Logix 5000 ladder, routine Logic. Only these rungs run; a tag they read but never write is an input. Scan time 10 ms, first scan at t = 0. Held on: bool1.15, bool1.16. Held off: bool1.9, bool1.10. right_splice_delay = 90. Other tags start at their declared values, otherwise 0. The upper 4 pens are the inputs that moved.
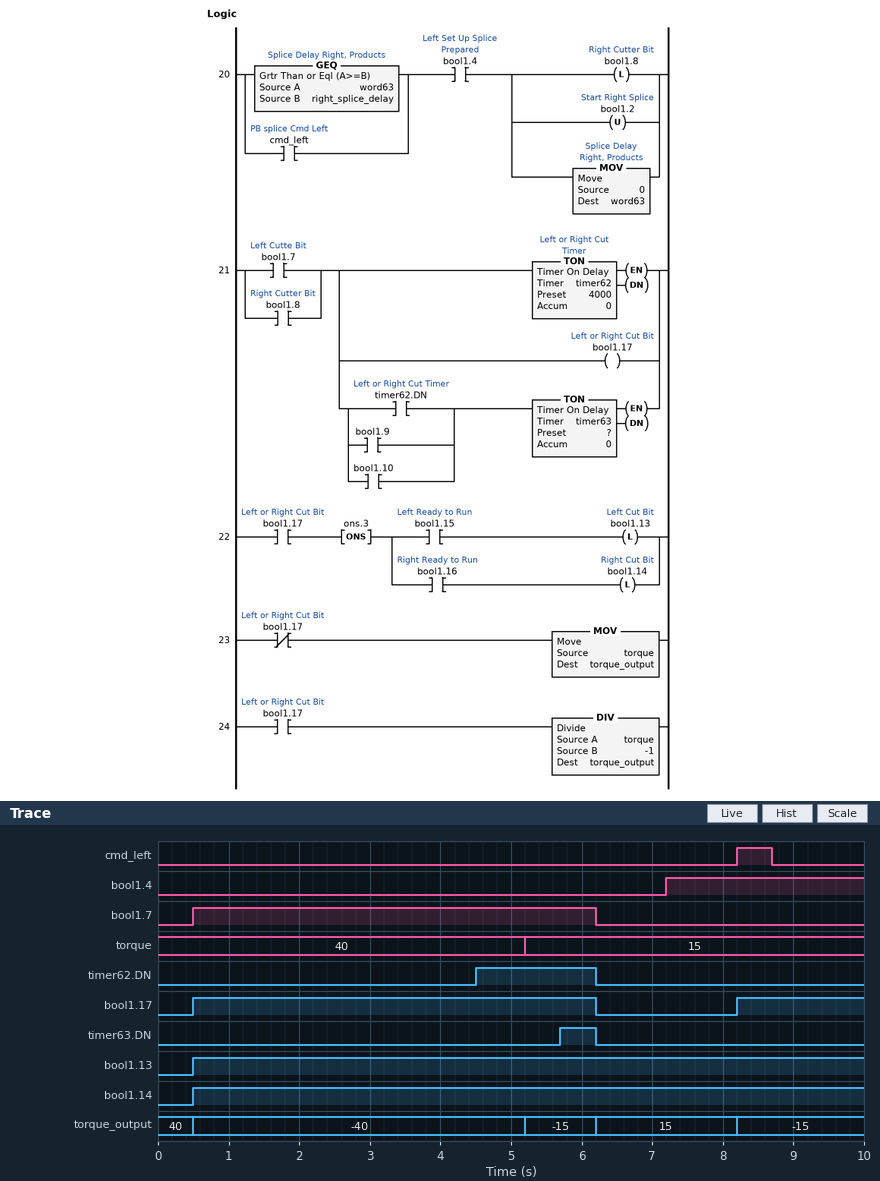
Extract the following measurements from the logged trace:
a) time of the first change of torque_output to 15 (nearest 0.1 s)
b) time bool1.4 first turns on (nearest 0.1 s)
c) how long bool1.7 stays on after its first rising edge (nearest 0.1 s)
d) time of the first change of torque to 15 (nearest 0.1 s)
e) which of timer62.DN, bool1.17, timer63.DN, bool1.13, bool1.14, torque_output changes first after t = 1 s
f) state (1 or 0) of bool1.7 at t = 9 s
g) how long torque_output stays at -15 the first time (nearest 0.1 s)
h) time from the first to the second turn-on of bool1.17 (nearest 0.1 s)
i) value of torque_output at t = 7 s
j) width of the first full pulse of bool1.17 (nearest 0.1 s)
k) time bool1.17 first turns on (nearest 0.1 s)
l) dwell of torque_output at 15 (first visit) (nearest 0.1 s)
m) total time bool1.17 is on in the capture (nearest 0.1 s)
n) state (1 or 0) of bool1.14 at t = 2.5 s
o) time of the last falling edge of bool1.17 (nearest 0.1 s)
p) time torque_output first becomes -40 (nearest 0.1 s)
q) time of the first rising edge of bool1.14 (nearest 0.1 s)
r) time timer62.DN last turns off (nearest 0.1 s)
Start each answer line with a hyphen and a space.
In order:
- 6.2 s
- 7.2 s
- 5.7 s
- 5.2 s
- timer62.DN
- 0
- 1.0 s
- 7.7 s
- 15
- 5.7 s
- 0.5 s
- 2.0 s
- 7.5 s
- 1
- 6.2 s
- 0.5 s
- 0.5 s
- 6.2 s
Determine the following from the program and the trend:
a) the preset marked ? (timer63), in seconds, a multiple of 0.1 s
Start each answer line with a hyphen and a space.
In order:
- 1.2 s
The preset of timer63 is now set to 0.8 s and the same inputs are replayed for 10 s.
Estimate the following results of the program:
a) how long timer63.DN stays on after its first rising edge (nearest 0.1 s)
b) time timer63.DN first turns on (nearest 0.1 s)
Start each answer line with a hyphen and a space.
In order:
- 0.9 s
- 5.3 s
